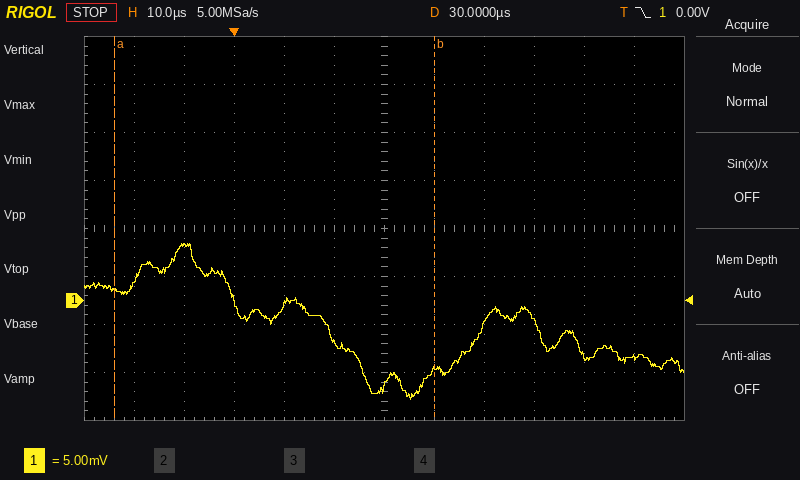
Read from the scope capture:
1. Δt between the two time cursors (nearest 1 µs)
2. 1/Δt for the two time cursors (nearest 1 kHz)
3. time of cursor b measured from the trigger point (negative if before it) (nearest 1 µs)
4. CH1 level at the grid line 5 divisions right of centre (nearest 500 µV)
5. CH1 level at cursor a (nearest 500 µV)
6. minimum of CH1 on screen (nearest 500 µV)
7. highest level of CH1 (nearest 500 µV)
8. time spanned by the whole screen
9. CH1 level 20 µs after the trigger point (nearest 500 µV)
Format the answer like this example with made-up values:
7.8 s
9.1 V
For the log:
64 µs
16 kHz
+40 µs
-6.0 mV
1.0 mV
-10.5 mV
6.0 mV
120 µs
-4.5 mV
